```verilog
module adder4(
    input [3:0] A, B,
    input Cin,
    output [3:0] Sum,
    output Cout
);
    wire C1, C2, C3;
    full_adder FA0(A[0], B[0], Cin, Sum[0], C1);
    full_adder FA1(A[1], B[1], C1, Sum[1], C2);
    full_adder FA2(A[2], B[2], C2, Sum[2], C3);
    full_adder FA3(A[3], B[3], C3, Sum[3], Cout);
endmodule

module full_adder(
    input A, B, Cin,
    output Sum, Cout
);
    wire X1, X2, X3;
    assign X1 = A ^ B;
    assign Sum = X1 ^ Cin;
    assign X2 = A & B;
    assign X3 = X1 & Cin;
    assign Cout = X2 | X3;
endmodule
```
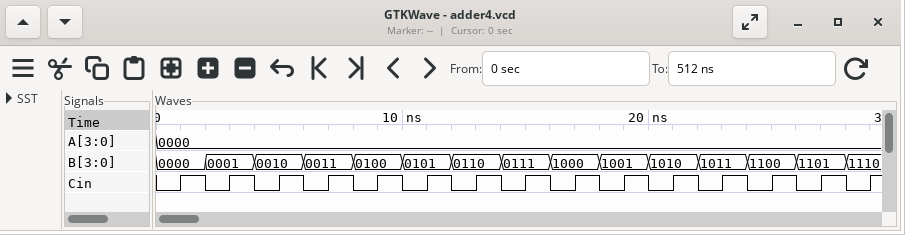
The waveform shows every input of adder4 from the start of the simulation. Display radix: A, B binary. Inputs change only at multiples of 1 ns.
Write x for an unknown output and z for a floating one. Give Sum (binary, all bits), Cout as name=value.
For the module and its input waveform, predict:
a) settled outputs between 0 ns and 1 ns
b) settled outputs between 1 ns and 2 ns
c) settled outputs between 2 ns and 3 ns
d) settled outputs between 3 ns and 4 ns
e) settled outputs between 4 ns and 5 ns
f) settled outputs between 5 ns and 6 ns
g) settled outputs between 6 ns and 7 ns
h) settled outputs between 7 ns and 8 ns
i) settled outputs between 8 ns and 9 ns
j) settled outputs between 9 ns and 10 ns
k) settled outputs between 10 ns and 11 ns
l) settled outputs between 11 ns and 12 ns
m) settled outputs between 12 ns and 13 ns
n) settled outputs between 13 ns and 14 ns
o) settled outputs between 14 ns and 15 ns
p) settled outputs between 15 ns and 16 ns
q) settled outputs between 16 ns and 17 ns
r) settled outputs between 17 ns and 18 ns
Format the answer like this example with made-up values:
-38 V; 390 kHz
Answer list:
Sum=0000, Cout=0; Sum=0001, Cout=0; Sum=0001, Cout=0; Sum=0010, Cout=0; Sum=0010, Cout=0; Sum=0011, Cout=0; Sum=0011, Cout=0; Sum=0100, Cout=0; Sum=0100, Cout=0; Sum=0101, Cout=0; Sum=0101, Cout=0; Sum=0110, Cout=0; Sum=0110, Cout=0; Sum=0111, Cout=0; Sum=0111, Cout=0; Sum=1000, Cout=0; Sum=1000, Cout=0; Sum=1001, Cout=0
